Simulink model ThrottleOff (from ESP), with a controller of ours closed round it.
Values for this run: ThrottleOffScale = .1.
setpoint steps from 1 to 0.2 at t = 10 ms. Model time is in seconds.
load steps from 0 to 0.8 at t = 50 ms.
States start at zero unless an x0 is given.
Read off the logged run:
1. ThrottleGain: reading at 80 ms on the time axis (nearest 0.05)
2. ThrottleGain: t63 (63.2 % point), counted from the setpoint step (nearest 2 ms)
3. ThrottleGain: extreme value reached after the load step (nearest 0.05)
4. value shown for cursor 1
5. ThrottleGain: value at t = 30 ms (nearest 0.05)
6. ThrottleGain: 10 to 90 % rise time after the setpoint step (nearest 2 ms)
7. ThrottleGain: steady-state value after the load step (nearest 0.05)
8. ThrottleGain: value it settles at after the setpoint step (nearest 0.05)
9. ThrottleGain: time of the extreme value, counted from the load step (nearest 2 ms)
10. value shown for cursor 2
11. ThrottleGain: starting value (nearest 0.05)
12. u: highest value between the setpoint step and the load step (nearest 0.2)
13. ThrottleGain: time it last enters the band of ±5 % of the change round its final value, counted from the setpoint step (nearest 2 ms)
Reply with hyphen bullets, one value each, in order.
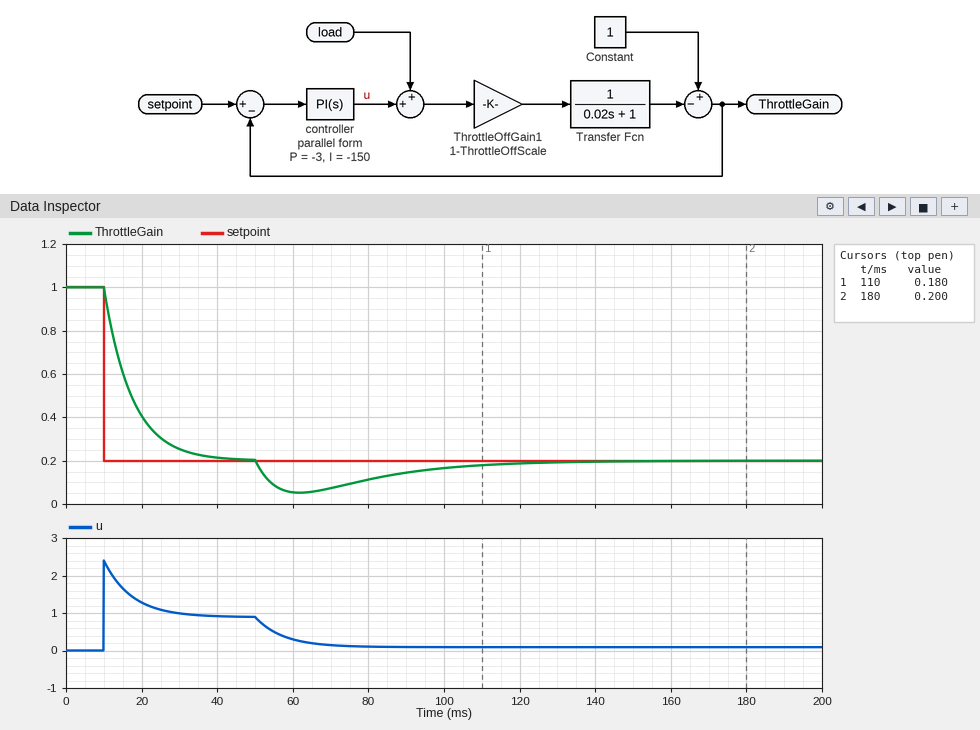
- 0.10
- 8 ms
- 0.05
- 0.180
- 0.25
- 16 ms
- 0.20
- 0.20
- 12 ms
- 0.200
- 1.00
- 2.4
- 22 ms
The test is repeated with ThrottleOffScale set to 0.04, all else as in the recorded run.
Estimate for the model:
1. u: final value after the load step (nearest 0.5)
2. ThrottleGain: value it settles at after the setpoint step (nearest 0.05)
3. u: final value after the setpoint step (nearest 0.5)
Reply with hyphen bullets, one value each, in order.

- 0.0
- 0.20
- 1.0
